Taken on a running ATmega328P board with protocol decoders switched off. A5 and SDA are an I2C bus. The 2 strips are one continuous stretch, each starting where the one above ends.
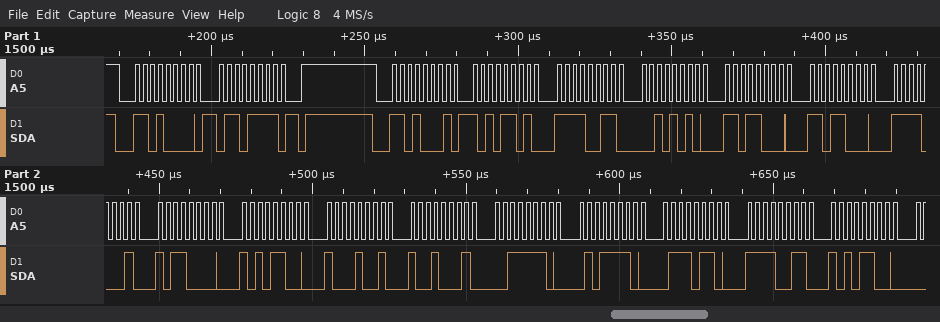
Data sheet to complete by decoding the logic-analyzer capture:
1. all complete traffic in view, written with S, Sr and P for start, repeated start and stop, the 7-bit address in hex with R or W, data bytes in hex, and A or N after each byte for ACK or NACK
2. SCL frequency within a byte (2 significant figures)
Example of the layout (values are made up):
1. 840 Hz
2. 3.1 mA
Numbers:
1. S 68W A 6F A P S 68R A AD A F3 A 2A A D8 A D8 A F1 A B0 A AC A 89 A 91 A 3E A 5E A 76 A F3 A AC A
2. 400 kHz
